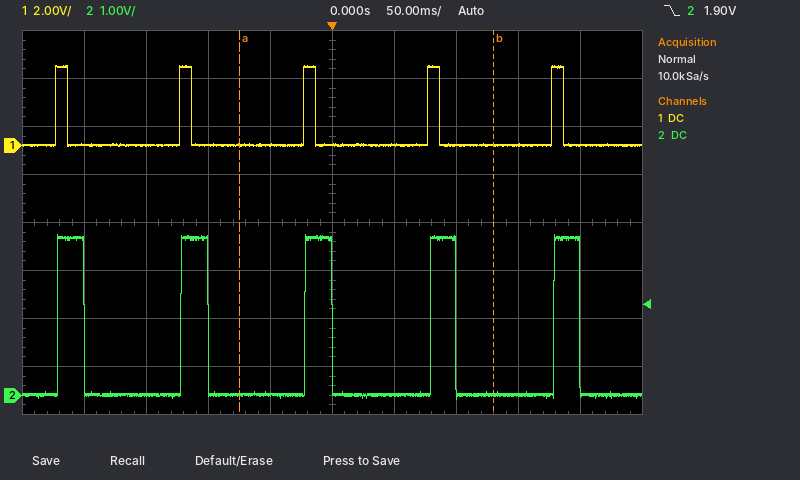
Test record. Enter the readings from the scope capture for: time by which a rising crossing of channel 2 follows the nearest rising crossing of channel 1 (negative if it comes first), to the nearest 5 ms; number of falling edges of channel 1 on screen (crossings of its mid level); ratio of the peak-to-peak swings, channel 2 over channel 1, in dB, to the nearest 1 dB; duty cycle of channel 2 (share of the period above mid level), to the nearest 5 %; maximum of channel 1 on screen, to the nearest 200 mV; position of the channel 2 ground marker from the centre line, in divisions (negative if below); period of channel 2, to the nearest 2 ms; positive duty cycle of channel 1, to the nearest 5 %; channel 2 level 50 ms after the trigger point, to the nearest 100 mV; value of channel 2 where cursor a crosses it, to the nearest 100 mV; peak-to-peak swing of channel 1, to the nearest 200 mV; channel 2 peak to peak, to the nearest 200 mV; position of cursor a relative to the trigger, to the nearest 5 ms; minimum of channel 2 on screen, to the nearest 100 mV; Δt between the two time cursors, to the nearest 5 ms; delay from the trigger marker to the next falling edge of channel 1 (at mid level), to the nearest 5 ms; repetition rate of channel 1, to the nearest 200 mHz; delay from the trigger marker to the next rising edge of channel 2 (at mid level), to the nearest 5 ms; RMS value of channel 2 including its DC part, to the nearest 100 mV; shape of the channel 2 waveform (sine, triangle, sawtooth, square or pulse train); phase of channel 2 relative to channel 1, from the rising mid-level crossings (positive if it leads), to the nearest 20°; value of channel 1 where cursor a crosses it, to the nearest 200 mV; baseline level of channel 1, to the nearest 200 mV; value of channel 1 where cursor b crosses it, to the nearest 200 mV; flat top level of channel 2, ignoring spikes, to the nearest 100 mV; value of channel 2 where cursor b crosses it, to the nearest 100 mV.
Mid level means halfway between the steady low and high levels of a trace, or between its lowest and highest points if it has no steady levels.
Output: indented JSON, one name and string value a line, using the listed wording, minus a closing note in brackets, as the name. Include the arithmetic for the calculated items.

{
  "time by which a rising crossing of channel 2 follows the nearest rising crossing of channel 1 (negative if it comes first), to the nearest 5 ms": "0 ms",
  "number of falling edges of channel 1 on screen": "5",
  "ratio of the peak-to-peak swings, channel 2 over channel 1, in dB, to the nearest 1 dB": "20 log10(3.4 V / 3.4 V) ≈ 0 dB",
  "duty cycle of channel 2 (share of the period above mid level), to the nearest 5 %": "20 %",
  "maximum of channel 1 on screen, to the nearest 200 mV": "3.4 V",
  "position of the channel 2 ground marker from the centre line, in divisions": "-3.6 div",
  "period of channel 2, to the nearest 2 ms": "100 ms",
  "positive duty cycle of channel 1, to the nearest 5 %": "10 %",
  "channel 2 level 50 ms after the trigger point, to the nearest 100 mV": "0.0 V",
  "value of channel 2 where cursor a crosses it, to the nearest 100 mV": "0.0 V",
  "peak-to-peak swing of channel 1, to the nearest 200 mV": "3.4 V − (0.0 V) = 3.4 V",
  "channel 2 peak to peak, to the nearest 200 mV": "3.4 V",
  "position of cursor a relative to the trigger, to the nearest 5 ms": "-75 ms",
  "minimum of channel 2 on screen, to the nearest 100 mV": "-100 mV",
  "Δt between the two time cursors, to the nearest 5 ms": "205 ms",
  "delay from the trigger marker to the next falling edge of channel 1 (at mid level), to the nearest 5 ms": "85 ms",
  "repetition rate of channel 1, to the nearest 200 mHz": "1 / 100 ms ≈ 10.0 Hz",
  "delay from the trigger marker to the next rising edge of channel 2 (at mid level), to the nearest 5 ms": "80 ms",
  "RMS value of channel 2 including its DC part, to the nearest 100 mV": "√(0.2 × (3.3 V)² + 0.8 × (-100 mV)²) ≈ 1.5 V",
  "shape of the channel 2 waveform": "pulse train",
  "phase of channel 2 relative to channel 1, from the rising mid-level crossings (positive if it leads), to the nearest 20°": "−360° × (0 ms) / 100 ms ≈ 0°",
  "value of channel 1 where cursor a crosses it, to the nearest 200 mV": "0.0 V",
  "baseline level of channel 1, to the nearest 200 mV": "0.0 V",
  "value of channel 1 where cursor b crosses it, to the nearest 200 mV": "0.0 V",
  "flat top level of channel 2, ignoring spikes, to the nearest 100 mV": "3.3 V",
  "value of channel 2 where cursor b crosses it, to the nearest 100 mV": "0.0 V"
}
